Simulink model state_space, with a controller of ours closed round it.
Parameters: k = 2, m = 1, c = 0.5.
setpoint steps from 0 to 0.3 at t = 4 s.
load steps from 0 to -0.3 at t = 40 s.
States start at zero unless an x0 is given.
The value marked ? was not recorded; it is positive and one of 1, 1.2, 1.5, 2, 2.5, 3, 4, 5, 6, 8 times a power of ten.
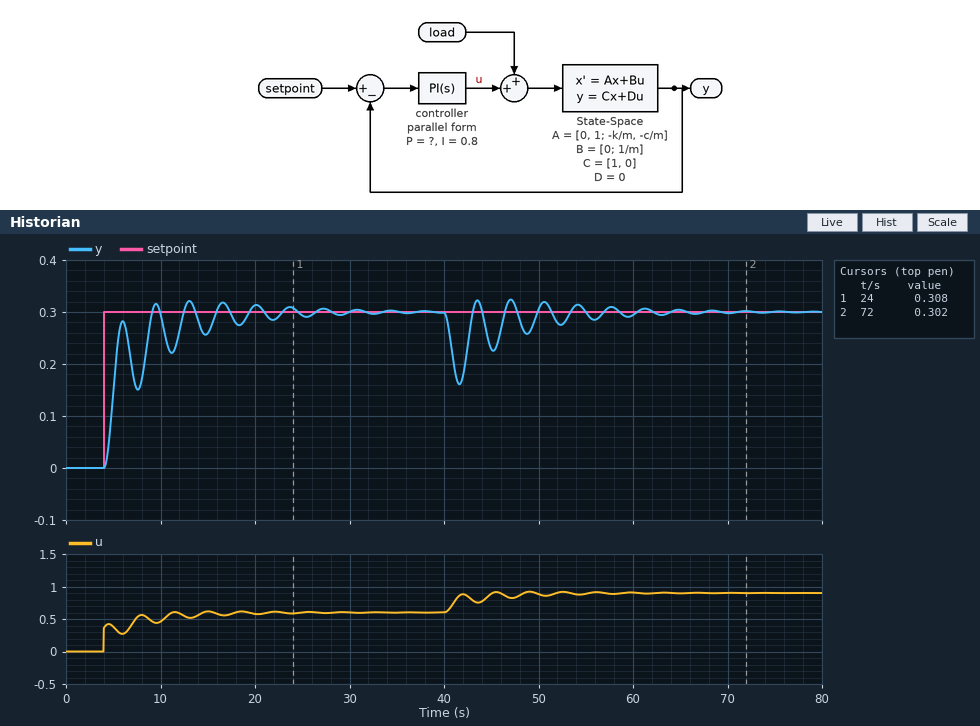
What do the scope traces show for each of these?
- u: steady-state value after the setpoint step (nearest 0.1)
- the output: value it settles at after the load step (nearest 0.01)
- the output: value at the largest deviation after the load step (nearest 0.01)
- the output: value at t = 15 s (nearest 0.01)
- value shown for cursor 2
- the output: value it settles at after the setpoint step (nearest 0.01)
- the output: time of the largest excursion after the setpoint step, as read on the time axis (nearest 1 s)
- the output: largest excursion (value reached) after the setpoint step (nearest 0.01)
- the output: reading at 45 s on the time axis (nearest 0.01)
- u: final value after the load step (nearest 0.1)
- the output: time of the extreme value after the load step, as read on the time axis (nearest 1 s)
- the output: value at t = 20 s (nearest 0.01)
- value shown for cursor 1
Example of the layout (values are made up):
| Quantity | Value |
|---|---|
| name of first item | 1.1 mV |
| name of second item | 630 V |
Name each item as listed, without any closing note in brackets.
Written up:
| Quantity | Value |
|---|---|
| u: steady-state value after the setpoint step | 0.6 |
| the output: value it settles at after the load step | 0.30 |
| the output: value at the largest deviation after the load step | 0.16 |
| the output: value at t = 15 s | 0.26 |
| value shown for cursor 2 | 0.302 |
| the output: value it settles at after the setpoint step | 0.30 |
| the output: time of the largest excursion after the setpoint step, as read on the time axis | 13 s |
| the output: largest excursion (value reached) after the setpoint step | 0.32 |
| the output: reading at 45 s on the time axis | 0.23 |
| u: final value after the load step | 0.9 |
| the output: time of the extreme value after the load step, as read on the time axis | 42 s |
| the output: value at t = 20 s | 0.31 |
| value shown for cursor 1 | 0.308 |
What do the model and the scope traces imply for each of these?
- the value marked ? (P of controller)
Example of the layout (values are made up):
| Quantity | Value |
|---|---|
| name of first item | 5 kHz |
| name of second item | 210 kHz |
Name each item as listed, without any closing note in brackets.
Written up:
| Quantity | Value |
|---|---|
| the value marked ? | 1.2 |
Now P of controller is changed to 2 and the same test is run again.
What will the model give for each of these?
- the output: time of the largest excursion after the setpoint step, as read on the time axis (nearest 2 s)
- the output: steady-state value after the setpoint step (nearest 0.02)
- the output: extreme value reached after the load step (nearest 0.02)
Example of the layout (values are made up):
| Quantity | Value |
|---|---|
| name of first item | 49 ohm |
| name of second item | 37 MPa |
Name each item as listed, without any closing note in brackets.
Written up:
| Quantity | Value |
|---|---|
| the output: time of the largest excursion after the setpoint step, as read on the time axis | 8 s |
| the output: steady-state value after the setpoint step | 0.30 |
| the output: extreme value reached after the load step | 0.18 |
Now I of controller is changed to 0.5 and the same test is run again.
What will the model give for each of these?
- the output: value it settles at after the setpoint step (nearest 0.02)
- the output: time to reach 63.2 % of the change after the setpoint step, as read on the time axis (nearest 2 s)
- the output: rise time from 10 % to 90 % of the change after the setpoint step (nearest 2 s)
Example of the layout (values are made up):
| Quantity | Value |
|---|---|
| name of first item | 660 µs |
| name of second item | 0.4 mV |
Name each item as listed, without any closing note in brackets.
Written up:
| Quantity | Value |
|---|---|
| the output: value it settles at after the setpoint step | 0.30 |
| the output: time to reach 63.2 % of the change after the setpoint step, as read on the time axis | 6 s |
| the output: rise time from 10 % to 90 % of the change after the setpoint step | 8 s |
